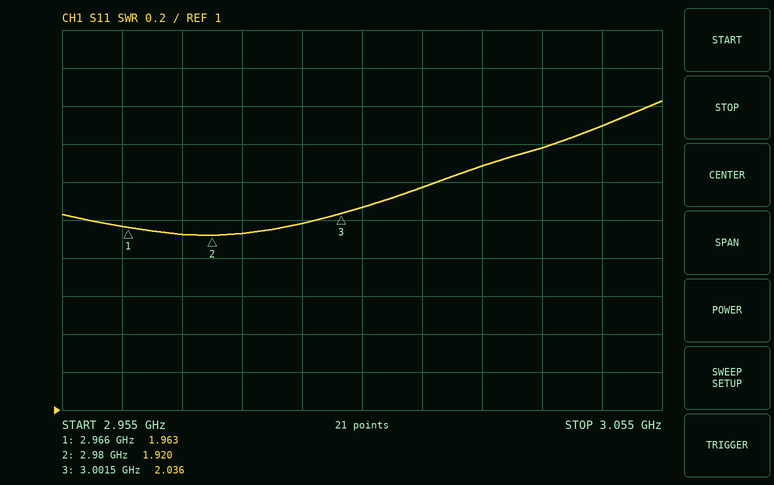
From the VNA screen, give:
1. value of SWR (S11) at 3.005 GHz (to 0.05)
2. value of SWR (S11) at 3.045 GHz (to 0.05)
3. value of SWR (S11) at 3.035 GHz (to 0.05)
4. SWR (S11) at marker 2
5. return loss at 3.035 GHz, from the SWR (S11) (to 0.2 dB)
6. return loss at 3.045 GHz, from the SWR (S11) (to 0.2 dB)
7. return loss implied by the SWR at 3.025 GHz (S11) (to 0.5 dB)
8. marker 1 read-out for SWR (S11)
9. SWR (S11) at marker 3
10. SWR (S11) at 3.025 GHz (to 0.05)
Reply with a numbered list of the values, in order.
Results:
1. 2.05
2. 2.50
3. 2.40
4. 1.920
5. 7.8 dB
6. 7.4 dB
7. 8.0 dB
8. 1.963
9. 2.036
10. 2.30
